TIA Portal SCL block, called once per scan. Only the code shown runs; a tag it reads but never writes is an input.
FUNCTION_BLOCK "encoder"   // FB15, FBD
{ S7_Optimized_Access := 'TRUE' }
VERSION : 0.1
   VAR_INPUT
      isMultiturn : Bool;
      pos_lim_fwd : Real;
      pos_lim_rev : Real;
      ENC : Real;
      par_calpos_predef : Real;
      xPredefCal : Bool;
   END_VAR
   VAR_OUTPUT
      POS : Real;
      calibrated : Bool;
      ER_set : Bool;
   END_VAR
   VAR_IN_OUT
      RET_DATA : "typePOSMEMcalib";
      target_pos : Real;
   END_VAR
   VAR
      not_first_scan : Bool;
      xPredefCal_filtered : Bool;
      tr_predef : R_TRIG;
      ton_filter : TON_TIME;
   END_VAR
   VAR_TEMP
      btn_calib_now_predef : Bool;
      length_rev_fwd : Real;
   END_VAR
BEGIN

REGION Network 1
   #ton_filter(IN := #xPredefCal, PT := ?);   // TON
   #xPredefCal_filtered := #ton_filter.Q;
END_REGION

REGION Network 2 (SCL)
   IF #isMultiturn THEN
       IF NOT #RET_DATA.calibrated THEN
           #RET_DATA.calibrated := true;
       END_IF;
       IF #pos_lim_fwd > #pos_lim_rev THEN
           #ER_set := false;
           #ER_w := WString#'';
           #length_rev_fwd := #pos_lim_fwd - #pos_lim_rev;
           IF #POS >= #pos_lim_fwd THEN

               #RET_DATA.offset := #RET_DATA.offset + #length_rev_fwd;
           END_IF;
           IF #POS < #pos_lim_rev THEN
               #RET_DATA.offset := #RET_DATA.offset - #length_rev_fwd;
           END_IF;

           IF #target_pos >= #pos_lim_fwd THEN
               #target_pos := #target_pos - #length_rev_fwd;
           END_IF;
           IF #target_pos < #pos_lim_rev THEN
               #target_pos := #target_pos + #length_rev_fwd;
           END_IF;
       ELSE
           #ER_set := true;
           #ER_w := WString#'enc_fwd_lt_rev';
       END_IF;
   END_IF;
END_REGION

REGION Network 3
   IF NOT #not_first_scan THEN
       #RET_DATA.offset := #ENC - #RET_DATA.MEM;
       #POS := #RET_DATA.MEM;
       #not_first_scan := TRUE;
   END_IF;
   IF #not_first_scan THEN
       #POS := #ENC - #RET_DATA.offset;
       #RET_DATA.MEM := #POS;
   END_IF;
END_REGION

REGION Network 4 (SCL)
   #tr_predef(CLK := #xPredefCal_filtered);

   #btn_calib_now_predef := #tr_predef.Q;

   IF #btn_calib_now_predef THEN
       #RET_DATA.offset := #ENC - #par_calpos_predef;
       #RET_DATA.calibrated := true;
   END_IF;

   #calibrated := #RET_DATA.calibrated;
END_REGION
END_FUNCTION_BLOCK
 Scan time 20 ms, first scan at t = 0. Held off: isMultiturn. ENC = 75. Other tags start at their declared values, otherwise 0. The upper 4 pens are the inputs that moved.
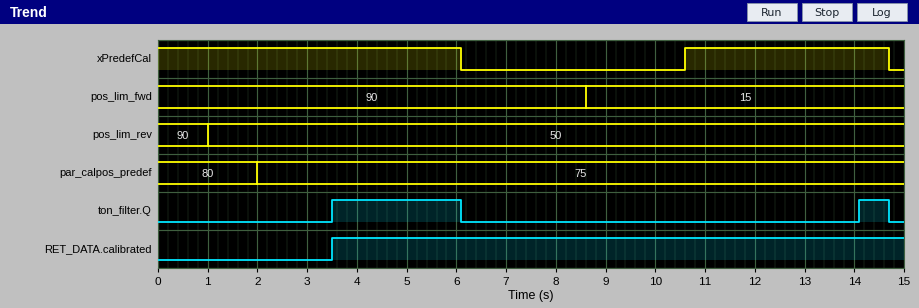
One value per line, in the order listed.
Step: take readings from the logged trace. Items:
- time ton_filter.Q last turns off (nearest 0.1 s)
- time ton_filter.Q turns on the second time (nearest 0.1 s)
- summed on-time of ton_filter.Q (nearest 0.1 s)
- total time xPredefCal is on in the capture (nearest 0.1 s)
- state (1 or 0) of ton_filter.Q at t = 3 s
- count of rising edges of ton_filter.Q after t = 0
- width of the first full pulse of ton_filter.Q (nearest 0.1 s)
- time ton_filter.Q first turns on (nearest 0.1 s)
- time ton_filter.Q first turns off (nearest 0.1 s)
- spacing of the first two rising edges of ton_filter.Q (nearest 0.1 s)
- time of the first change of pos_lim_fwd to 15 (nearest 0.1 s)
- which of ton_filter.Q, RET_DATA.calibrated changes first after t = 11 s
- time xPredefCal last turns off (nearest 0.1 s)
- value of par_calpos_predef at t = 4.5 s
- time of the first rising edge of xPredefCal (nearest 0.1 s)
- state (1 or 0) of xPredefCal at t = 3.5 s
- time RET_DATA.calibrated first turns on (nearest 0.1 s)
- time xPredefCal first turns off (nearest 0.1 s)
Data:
14.7 s
14.1 s
3.2 s
10.2 s
0
2
2.6 s
3.5 s
6.1 s
10.6 s
8.6 s
ton_filter.Q
14.7 s
75
10.6 s
1
3.5 s
6.1 s
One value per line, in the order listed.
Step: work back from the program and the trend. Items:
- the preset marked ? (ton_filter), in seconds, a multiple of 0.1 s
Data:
3.5 s
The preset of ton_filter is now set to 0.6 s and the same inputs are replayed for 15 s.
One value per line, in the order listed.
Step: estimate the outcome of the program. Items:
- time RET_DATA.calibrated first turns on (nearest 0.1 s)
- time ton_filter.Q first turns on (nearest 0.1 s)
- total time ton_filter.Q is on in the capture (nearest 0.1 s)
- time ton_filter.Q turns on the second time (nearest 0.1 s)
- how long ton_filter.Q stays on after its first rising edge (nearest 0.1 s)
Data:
0.6 s
0.6 s
9.0 s
11.2 s
5.5 s
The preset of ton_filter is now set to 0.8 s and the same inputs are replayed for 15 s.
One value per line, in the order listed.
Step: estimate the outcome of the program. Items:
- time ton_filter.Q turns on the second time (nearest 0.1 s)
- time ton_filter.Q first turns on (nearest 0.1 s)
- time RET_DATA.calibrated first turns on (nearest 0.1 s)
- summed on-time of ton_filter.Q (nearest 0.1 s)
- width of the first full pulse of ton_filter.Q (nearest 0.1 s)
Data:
11.4 s
0.8 s
0.8 s
8.6 s
5.3 s
